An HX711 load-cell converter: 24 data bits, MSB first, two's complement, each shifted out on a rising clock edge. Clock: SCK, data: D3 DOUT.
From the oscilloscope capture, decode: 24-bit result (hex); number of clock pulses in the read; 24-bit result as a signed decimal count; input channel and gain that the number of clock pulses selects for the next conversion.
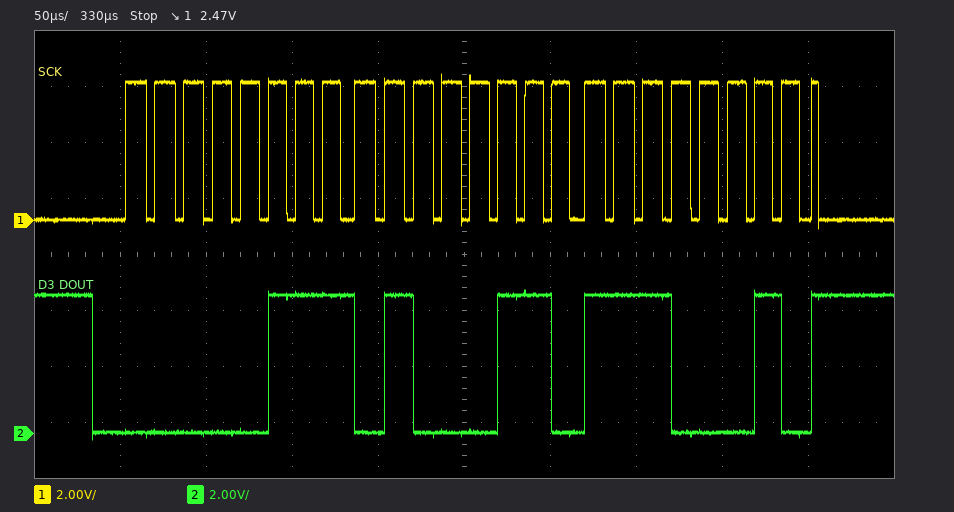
0x0746E2
25
476898
channel A, gain 128
